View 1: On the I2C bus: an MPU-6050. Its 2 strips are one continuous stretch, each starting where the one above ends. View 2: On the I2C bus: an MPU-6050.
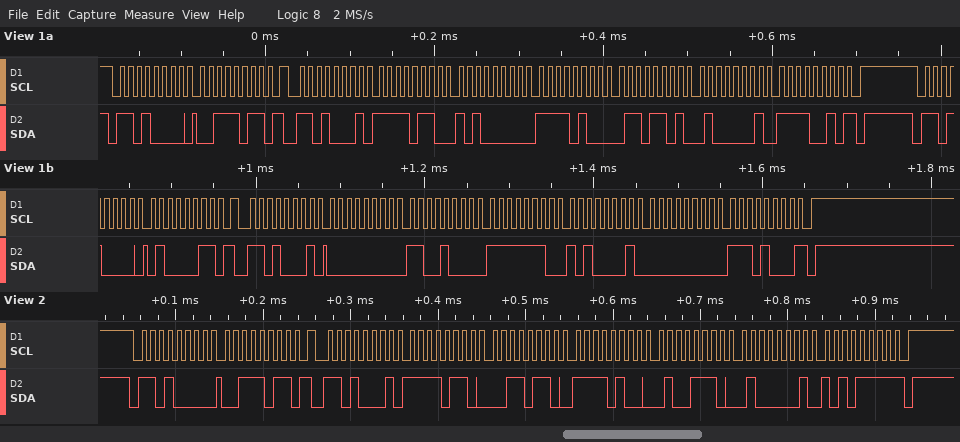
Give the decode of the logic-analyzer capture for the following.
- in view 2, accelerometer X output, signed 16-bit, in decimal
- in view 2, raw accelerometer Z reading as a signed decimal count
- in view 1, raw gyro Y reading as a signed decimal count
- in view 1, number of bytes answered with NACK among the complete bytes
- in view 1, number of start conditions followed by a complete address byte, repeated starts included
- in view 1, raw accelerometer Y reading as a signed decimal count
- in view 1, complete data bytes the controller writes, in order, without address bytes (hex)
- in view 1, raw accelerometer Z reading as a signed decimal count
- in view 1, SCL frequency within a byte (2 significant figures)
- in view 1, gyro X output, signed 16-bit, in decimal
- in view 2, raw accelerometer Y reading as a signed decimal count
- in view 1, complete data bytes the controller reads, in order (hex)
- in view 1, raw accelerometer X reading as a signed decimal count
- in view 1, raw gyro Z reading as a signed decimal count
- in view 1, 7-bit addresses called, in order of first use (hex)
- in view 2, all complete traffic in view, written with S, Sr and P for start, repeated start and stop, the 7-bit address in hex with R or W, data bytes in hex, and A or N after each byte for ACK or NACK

-2506
16815
-351
2
4
-2963
3B 43
16882
100 kHz
200
-2994
F6 A0 F4 6D 41 F2 00 C8 FE A1 00 E8
-2400
232
0x68
S 68W A 3B A Sr 68R A F6 A 36 A F4 A 4E A 41 A AF N P
